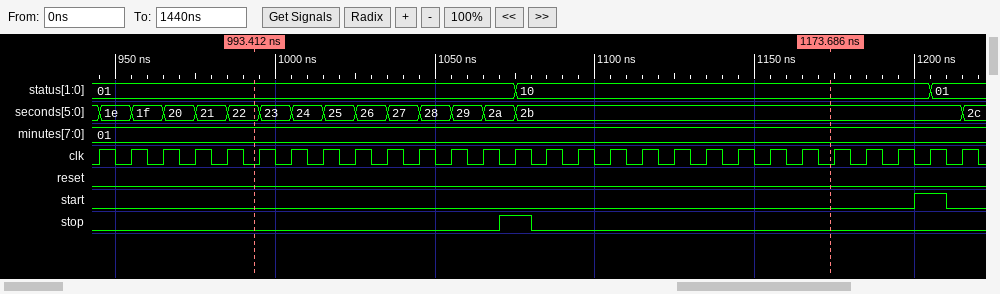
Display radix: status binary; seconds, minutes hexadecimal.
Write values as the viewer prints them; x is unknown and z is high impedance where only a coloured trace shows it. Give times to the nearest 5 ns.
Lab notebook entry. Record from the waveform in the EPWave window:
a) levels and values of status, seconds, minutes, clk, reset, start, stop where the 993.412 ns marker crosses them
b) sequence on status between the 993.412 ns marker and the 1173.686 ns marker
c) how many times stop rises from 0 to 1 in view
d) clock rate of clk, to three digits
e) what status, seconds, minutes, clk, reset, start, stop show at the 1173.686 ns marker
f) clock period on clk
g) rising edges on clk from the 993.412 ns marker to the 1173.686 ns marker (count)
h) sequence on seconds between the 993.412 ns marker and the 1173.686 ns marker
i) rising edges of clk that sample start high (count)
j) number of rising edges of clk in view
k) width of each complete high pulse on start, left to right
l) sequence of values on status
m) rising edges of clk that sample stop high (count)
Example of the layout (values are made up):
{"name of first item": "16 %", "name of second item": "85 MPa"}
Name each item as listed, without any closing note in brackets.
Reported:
{"levels and values of status, seconds, minutes, clk, reset, start, stop where the 993.412 ns marker crosses them": "status=01, seconds=22, minutes=01, clk=0, reset=0, start=0, stop=0", "sequence on status between the 993.412 ns marker and the 1173.686 ns marker": "01, 10", "how many times stop rises from 0 to 1 in view": "1", "clock rate of clk, to three digits": "100 MHz", "what status, seconds, minutes, clk, reset, start, stop show at the 1173.686 ns marker": "status=10, seconds=2b, minutes=01, clk=0, reset=0, start=0, stop=0", "clock period on clk": "10 ns", "rising edges on clk from the 993.412 ns marker to the 1173.686 ns marker": "18", "sequence on seconds between the 993.412 ns marker and the 1173.686 ns marker": "22, 23, 24, 25, 26, 27, 28, 29, 2a, 2b", "rising edges of clk that sample start high": "1", "number of rising edges of clk in view": "28", "width of each complete high pulse on start, left to right": "10 ns", "sequence of values on status": "01, 10, 01", "rising edges of clk that sample stop high": "1"}
